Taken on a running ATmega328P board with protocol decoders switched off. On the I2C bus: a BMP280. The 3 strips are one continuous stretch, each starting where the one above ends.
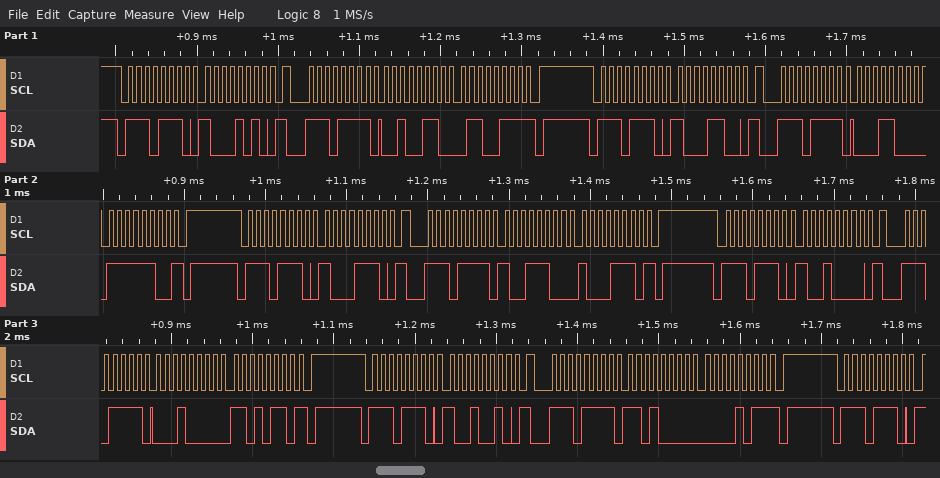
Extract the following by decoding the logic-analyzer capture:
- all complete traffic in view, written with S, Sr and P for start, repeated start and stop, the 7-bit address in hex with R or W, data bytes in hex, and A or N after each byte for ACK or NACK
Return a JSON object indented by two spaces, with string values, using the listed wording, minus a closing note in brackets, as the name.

{
  "all complete traffic in view, written with S, Sr and P for start, repeated start and stop, the 7-bit address in hex with R or W, data bytes in hex, and A or N after each byte for ACK or NACK": "S 77W A 8A A Sr 77R A 26 A 67 N P S 77W A 8C A Sr 77R A 18 A FC N P S 77W A 8E A Sr 77R A 9C A 8E N P S 77W A 90 A Sr 77R A 10 A D6 N P S 77W A 92 A Sr 77R A D0 A 0B N P S 77W A"
}
